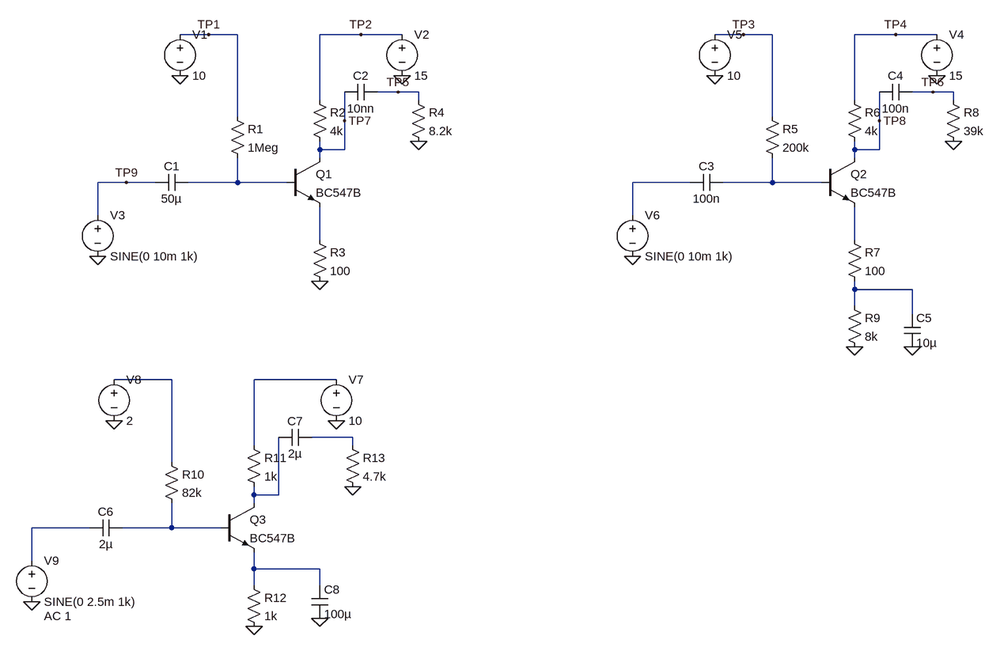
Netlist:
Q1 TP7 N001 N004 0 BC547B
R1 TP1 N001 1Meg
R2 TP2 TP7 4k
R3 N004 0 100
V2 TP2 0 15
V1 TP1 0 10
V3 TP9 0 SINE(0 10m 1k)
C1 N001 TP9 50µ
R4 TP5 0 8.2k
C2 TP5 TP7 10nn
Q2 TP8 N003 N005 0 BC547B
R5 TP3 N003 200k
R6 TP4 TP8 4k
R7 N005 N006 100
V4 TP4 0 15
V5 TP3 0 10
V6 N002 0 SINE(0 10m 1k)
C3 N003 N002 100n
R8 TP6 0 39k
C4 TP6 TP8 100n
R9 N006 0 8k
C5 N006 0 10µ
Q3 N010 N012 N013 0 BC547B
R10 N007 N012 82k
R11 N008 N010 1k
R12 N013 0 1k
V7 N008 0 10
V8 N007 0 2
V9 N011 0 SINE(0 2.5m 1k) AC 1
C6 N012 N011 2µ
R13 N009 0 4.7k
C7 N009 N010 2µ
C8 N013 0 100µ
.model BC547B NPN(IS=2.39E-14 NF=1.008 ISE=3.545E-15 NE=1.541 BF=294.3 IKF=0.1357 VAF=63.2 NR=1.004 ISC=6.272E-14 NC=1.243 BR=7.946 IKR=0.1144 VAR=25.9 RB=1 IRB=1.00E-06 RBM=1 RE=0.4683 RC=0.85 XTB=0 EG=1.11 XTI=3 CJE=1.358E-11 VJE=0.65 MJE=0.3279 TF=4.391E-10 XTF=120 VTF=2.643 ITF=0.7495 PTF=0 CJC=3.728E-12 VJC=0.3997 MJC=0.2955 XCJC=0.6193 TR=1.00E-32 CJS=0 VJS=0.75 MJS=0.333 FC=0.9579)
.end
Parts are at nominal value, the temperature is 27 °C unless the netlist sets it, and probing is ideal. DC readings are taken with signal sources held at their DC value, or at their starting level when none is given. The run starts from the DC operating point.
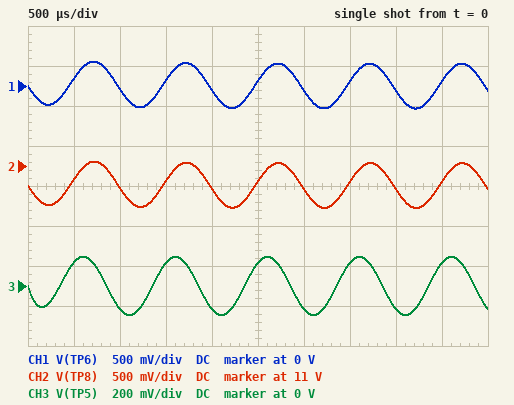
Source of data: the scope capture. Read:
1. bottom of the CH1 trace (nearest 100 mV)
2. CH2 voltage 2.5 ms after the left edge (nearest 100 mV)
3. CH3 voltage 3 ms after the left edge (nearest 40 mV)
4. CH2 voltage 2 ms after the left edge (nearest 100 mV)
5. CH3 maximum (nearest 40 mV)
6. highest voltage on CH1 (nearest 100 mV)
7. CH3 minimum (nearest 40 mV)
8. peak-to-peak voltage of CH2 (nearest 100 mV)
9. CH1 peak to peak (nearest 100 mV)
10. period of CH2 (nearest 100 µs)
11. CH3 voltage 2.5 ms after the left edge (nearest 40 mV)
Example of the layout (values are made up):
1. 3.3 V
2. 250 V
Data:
1. -300 mV
2. 10.8 V
3. -120 mV
4. 10.7 V
5. 160 mV
6. 300 mV
7. -160 mV
8. 600 mV
9. 600 mV
10. 1.0 ms
11. 120 mV
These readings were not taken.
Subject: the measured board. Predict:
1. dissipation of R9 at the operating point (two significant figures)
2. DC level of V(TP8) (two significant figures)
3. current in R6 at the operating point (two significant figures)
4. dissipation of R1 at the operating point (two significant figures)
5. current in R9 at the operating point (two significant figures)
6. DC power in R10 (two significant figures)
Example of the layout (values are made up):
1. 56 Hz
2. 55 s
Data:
1. 9.1 mW
2. 11 V
3. 1.1 mA
4. 82 µW
5. 1.1 mA
6. 960 nW
